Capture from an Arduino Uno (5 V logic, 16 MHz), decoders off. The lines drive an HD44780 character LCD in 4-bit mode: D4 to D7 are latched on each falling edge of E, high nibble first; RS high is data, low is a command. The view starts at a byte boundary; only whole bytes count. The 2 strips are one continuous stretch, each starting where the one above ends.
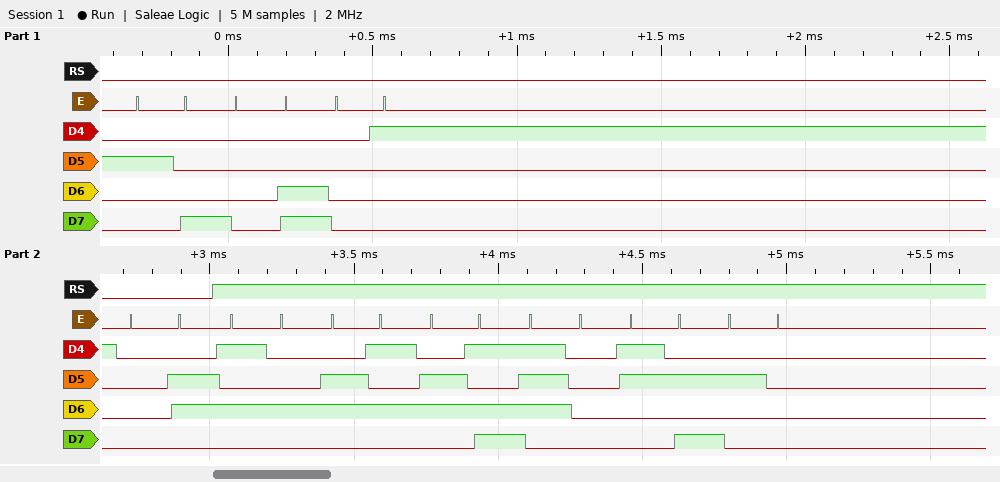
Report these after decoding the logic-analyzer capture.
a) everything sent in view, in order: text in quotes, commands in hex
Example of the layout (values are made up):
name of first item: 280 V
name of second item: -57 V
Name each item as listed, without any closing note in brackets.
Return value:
everything sent in view, in order: text in quotes, commands in hex: 0x28 0x0C 0x01 0x06 "Temp: "
